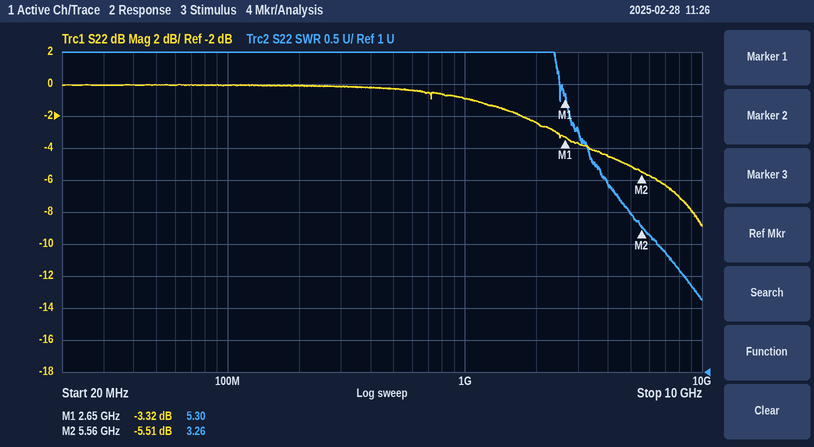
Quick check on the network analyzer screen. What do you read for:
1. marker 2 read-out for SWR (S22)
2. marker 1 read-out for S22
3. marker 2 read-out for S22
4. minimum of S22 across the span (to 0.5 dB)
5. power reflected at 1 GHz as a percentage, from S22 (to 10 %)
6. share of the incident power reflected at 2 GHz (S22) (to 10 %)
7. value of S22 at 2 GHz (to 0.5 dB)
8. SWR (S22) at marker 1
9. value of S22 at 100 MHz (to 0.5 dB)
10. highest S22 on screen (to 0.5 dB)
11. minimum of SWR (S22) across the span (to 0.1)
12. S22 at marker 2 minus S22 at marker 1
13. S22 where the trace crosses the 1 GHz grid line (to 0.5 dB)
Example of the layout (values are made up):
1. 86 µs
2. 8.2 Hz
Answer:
1. 3.26
2. -3.32 dB
3. -5.51 dB
4. -9.0 dB
5. 80 %
6. 60 %
7. -2.5 dB
8. 5.30
9. 0.0 dB
10. 0.0 dB
11. 2.1
12. -2.19 dB
13. -1.0 dB
